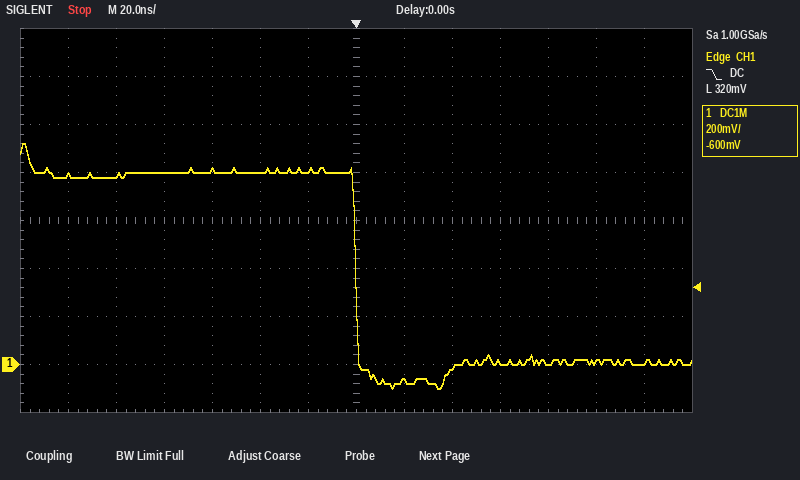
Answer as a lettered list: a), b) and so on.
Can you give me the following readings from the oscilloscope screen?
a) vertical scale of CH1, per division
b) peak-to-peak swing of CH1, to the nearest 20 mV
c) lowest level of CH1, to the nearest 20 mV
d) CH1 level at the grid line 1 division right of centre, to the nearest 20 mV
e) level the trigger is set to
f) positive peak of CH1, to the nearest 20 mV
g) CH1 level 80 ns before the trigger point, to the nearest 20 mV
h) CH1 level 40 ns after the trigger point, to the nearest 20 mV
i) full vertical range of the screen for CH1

a) 200 mV
b) 1.02 V
c) -100 mV
d) -60 mV
e) 320 mV
f) 920 mV
g) 800 mV
h) -20 mV
i) 1.6 V
